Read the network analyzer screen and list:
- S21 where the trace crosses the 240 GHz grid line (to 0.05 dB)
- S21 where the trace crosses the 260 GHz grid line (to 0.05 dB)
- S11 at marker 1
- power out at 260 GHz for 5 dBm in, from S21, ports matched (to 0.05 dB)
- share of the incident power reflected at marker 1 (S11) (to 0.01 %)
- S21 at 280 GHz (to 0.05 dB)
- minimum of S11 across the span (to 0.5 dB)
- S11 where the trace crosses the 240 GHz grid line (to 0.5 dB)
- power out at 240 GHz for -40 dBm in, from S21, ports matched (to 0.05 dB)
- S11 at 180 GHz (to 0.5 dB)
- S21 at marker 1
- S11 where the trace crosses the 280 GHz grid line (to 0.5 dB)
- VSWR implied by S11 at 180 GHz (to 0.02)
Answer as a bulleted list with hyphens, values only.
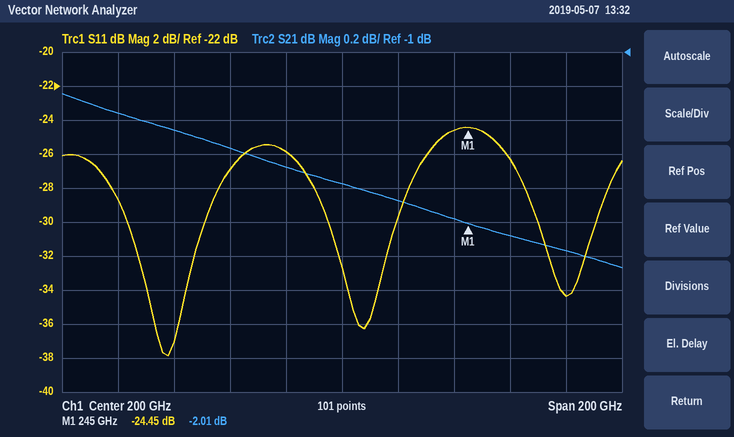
- -2.00 dB
- -2.10 dB
- -24.45 dB
- 2.90 dBm
- 0.36 %
- -2.15 dB
- -38.0 dB
- -24.5 dB
- -42.00 dBm
- -26.0 dB
- -2.01 dB
- -34.5 dB
- 1.10
